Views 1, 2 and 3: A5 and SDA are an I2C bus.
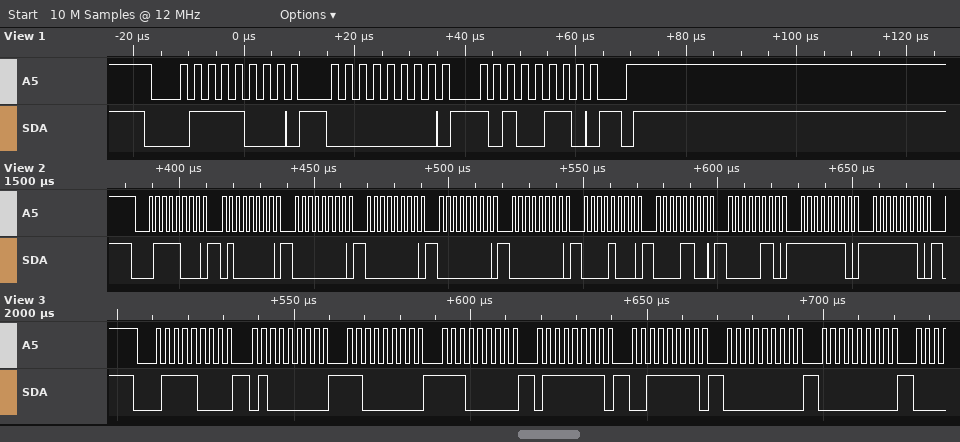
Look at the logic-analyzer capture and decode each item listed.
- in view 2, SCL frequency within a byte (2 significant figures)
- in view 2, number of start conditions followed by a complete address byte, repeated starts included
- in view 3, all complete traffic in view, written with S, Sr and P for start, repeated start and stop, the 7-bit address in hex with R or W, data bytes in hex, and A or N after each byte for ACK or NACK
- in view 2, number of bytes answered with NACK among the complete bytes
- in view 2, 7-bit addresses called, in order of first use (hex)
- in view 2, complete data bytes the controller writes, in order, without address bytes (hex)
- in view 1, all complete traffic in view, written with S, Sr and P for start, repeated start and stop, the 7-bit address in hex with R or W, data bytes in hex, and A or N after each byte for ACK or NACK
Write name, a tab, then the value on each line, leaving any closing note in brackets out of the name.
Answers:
in view 2, SCL frequency within a byte	400 kHz
in view 2, number of start conditions followed by a complete address byte, repeated starts included	1
in view 3, all complete traffic in view, written with S, Sr and P for start, repeated start and stop, the 7-bit address in hex with R or W, data bytes in hex, and A or N after each byte for ACK or NACK	S 3CW A 40 A C0 A E0 A 7F A 3F A 00 A 00 A
in view 2, number of bytes answered with NACK among the complete bytes	0
in view 2, 7-bit addresses called, in order of first use	0x3C
in view 2, complete data bytes the controller writes, in order, without address bytes	40 00 00 00 00 08 0C 06 FE FE
in view 1, all complete traffic in view, written with S, Sr and P for start, repeated start and stop, the 7-bit address in hex with R or W, data bytes in hex, and A or N after each byte for ACK or NACK	S 3CW A 00 A A6 A P
